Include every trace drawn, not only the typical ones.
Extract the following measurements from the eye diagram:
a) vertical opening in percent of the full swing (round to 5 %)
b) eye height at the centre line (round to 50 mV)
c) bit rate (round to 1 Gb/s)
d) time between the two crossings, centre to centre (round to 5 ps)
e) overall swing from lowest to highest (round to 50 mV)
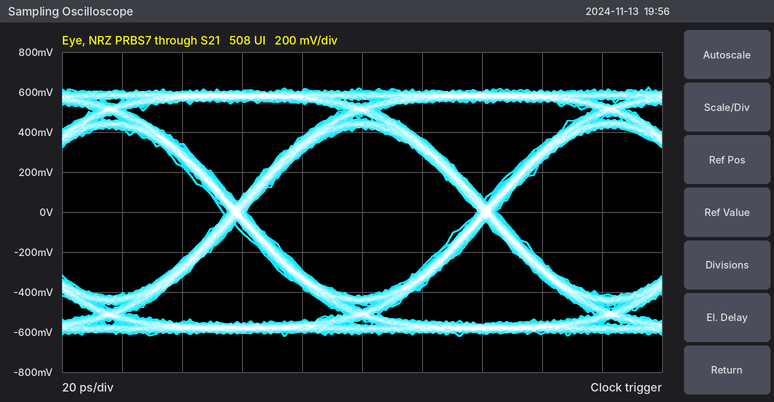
70 %
850 mV
12 Gb/s
85 ps
1.25 V
